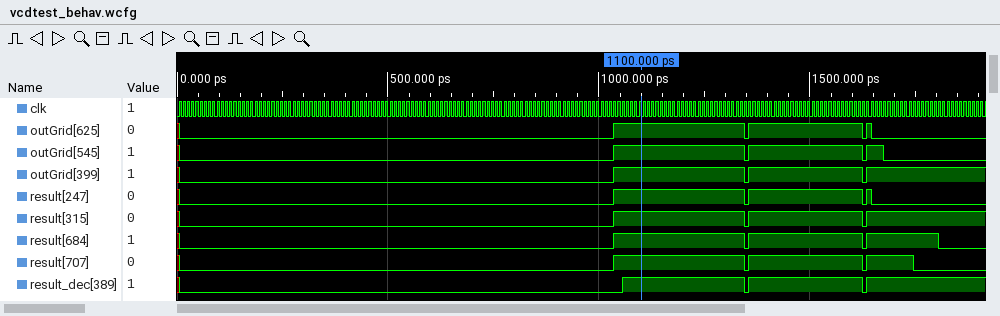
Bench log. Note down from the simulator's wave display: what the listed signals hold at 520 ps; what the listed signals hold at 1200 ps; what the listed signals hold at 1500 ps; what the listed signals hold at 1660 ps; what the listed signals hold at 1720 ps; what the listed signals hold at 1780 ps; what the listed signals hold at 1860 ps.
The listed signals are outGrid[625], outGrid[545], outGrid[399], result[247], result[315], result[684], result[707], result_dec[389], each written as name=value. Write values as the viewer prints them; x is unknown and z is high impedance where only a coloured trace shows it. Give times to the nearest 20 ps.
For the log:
outGrid[625]=0, outGrid[545]=0, outGrid[399]=0, result[247]=0, result[315]=0, result[684]=0, result[707]=0, result_dec[389]=0
outGrid[625]=1, outGrid[545]=1, outGrid[399]=1, result[247]=1, result[315]=1, result[684]=1, result[707]=1, result_dec[389]=1
outGrid[625]=1, outGrid[545]=1, outGrid[399]=1, result[247]=1, result[315]=1, result[684]=1, result[707]=1, result_dec[389]=1
outGrid[625]=0, outGrid[545]=1, outGrid[399]=1, result[247]=0, result[315]=1, result[684]=1, result[707]=1, result_dec[389]=1
outGrid[625]=0, outGrid[545]=0, outGrid[399]=1, result[247]=0, result[315]=1, result[684]=1, result[707]=1, result_dec[389]=1
outGrid[625]=0, outGrid[545]=0, outGrid[399]=1, result[247]=0, result[315]=1, result[684]=1, result[707]=0, result_dec[389]=1
outGrid[625]=0, outGrid[545]=0, outGrid[399]=1, result[247]=0, result[315]=1, result[684]=0, result[707]=0, result_dec[389]=1
